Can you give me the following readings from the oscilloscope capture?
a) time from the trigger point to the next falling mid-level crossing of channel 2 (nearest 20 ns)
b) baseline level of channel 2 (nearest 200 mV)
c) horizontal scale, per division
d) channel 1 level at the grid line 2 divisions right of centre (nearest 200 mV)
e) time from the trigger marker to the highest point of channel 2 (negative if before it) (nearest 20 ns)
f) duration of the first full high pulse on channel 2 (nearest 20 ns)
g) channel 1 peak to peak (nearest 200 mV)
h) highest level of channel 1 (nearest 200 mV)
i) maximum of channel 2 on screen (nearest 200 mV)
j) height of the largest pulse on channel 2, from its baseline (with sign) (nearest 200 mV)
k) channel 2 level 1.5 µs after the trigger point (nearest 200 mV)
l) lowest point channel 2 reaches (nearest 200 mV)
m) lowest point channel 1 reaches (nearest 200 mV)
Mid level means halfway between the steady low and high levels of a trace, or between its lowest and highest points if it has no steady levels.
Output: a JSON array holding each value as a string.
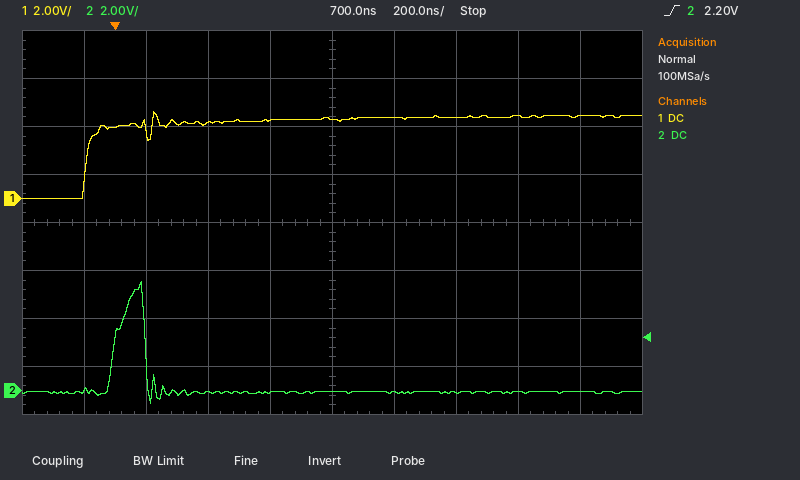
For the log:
["100 ns", "0.0 V", "200 ns", "3.4 V", "+80 ns", "100 ns", "3.6 V", "3.6 V", "4.6 V", "+4.6 V", "0.0 V", "-600 mV", "0.0 V"]
